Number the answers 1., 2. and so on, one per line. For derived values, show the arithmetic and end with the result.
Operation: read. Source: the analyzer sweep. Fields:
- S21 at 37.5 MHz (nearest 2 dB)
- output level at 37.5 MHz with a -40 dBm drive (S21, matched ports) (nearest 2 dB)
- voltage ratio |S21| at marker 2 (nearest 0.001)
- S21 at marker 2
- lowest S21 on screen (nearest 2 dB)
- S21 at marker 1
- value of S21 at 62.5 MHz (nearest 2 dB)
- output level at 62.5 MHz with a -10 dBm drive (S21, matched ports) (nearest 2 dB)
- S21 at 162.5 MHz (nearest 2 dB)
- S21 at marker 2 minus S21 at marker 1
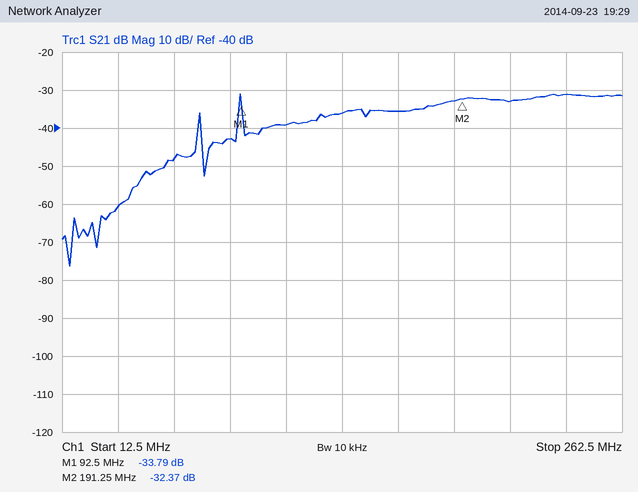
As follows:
1. -60 dB
2. -40 dBm + (-60 dB) = -100 dBm
3. 10^(-32.37/20) ≈ 0.024
4. -32.37 dB
5. -76 dB
6. -33.79 dB
7. -48 dB
8. -10 dBm + (-48 dB) = -58 dBm
9. -36 dB
10. -32.37 − (-33.79) = 1.42 dB
